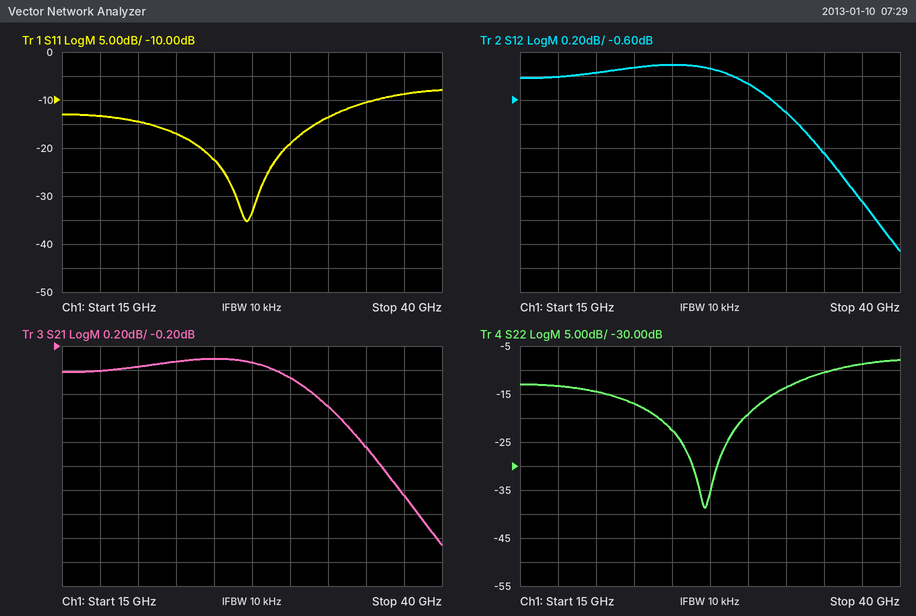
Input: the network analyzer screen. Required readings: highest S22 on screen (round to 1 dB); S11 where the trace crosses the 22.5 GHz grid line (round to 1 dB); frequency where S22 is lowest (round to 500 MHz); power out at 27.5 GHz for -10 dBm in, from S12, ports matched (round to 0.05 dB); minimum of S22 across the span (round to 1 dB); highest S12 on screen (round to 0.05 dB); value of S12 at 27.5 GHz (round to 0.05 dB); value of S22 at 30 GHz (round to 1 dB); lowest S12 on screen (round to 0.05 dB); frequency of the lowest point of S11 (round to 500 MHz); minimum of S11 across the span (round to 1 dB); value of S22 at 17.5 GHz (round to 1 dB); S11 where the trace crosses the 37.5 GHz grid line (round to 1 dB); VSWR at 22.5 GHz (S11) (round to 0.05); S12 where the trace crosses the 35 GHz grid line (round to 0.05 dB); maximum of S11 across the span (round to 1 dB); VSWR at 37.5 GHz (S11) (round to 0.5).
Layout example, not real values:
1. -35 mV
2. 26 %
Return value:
1. -8 dB
2. -17 dB
3. 27.0 GHz
4. -10.35 dBm
5. -39 dB
6. -0.30 dB
7. -0.35 dB
8. -19 dB
9. -1.85 dB
10. 27.0 GHz
11. -35 dB
12. -13 dB
13. -9 dB
14. 1.35
15. -1.05 dB
16. -8 dB
17. 2.0
